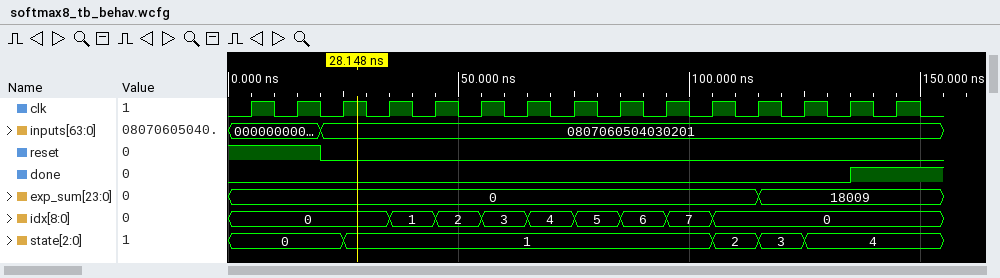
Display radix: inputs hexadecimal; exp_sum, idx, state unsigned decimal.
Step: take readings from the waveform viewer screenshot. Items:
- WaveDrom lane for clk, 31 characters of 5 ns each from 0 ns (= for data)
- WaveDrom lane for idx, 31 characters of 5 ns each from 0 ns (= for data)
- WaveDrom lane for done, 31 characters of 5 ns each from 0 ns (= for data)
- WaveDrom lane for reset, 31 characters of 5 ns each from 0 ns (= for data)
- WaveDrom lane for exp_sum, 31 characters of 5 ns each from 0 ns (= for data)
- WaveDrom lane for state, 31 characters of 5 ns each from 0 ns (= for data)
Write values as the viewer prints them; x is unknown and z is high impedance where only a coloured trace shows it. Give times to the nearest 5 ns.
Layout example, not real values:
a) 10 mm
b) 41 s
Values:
a) {name: 'clk', wave: '0101010101010101010101010101010'}
b) {name: 'idx', wave: '=......=.=.=.=.=.=.=.=.........', data: '0 1 2 3 4 5 6 7 0'}
c) {name: 'done', wave: '0..........................1...'}
d) {name: 'reset', wave: '1...0..........................'}
e) {name: 'exp_sum', wave: '=......................=.......', data: '0 18009'}
f) {name: 'state', wave: '=....=...............=.=.=.....', data: '0 1 2 3 4'}
